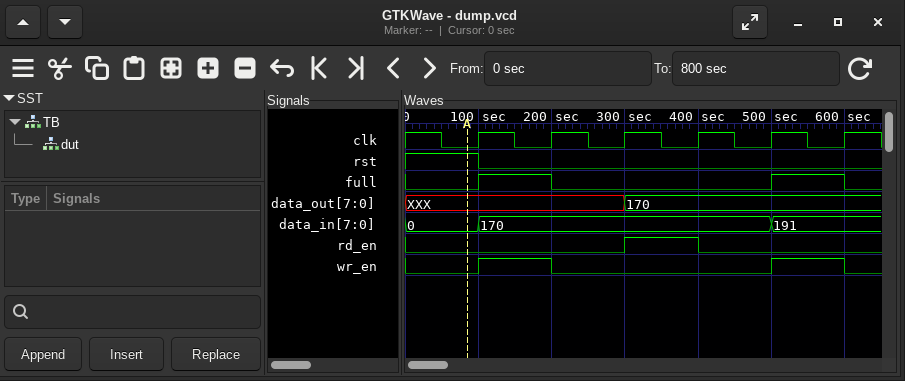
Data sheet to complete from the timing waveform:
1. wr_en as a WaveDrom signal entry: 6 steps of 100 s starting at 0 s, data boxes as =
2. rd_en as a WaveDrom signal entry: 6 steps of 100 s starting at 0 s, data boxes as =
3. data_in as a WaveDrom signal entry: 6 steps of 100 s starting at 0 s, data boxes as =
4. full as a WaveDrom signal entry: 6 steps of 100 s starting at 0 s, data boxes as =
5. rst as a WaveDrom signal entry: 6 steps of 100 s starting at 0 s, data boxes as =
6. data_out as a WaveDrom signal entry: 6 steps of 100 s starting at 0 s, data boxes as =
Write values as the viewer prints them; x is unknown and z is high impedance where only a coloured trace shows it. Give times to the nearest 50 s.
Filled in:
{name: 'wr_en', wave: '010..1'}
{name: 'rd_en', wave: '0..10.'}
{name: 'data_in', wave: '==...=', data: '0 170 191'}
{name: 'full', wave: '010..1'}
{name: 'rst', wave: '10....'}
{name: 'data_out', wave: 'x..=..', data: '170'}
